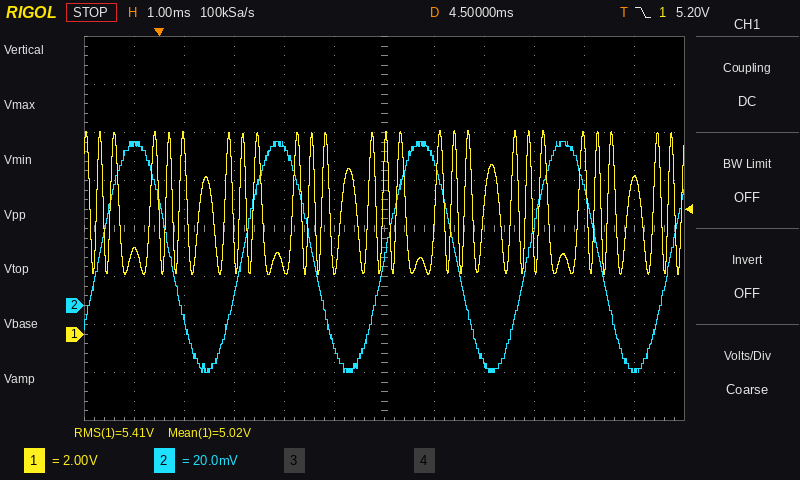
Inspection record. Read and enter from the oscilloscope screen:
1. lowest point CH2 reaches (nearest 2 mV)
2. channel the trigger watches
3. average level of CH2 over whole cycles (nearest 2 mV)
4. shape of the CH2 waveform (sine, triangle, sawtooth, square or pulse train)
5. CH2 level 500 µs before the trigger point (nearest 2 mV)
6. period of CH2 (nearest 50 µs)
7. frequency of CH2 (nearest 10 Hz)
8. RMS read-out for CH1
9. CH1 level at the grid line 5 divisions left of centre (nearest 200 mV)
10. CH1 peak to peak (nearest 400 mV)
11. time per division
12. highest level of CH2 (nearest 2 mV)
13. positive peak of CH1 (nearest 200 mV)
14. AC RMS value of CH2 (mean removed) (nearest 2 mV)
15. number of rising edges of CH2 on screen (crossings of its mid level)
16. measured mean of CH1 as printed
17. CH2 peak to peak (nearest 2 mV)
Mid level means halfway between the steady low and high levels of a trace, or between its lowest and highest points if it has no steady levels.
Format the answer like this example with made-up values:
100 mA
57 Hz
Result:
-28 mV
CH1
20 mV
sine
68 mV
2.85 ms
350 Hz
5.41 V
3.4 V
6.0 V
1 ms
68 mV
8.4 V
34 mV
5
5.02 V
96 mV
